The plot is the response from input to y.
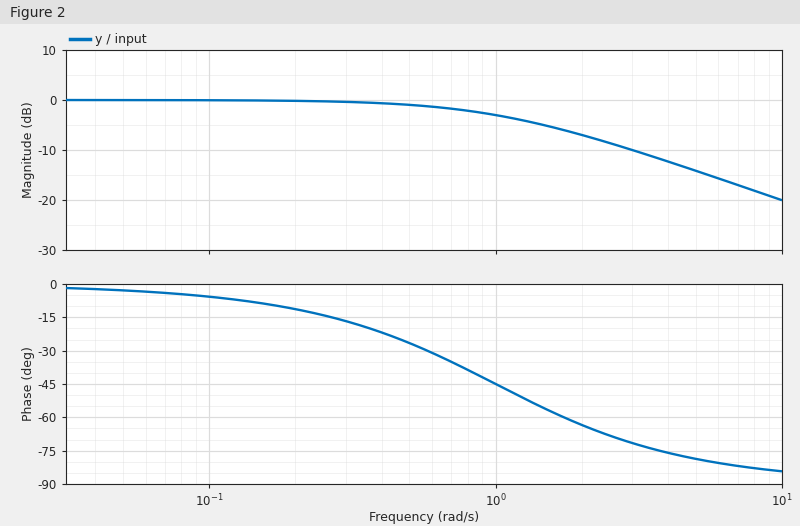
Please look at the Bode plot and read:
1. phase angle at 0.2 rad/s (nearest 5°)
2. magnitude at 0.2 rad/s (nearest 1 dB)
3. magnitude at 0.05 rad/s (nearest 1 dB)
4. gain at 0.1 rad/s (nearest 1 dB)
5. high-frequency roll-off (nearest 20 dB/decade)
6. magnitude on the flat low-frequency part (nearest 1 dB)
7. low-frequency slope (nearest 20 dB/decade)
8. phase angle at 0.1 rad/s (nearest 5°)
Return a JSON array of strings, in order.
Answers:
["-10°", "0 dB", "0 dB", "0 dB", "-20 dB/decade", "0 dB", "0 dB/decade", "-5°"]
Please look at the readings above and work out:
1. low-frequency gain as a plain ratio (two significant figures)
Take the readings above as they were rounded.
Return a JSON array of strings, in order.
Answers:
["1.0"]
